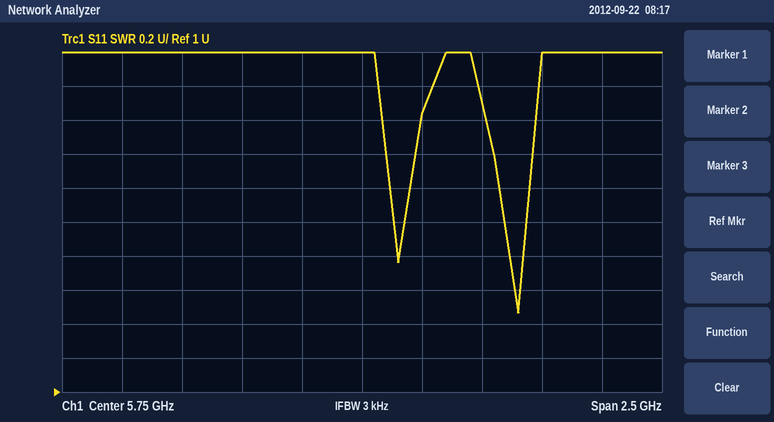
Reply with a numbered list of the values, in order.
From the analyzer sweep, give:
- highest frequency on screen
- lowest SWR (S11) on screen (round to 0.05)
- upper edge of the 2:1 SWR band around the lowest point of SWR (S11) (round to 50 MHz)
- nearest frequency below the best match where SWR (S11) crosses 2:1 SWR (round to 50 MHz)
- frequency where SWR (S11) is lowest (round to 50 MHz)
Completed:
1. 7 GHz
2. 1.45
3. 6.45 GHz
4. 6.35 GHz
5. 6.40 GHz
